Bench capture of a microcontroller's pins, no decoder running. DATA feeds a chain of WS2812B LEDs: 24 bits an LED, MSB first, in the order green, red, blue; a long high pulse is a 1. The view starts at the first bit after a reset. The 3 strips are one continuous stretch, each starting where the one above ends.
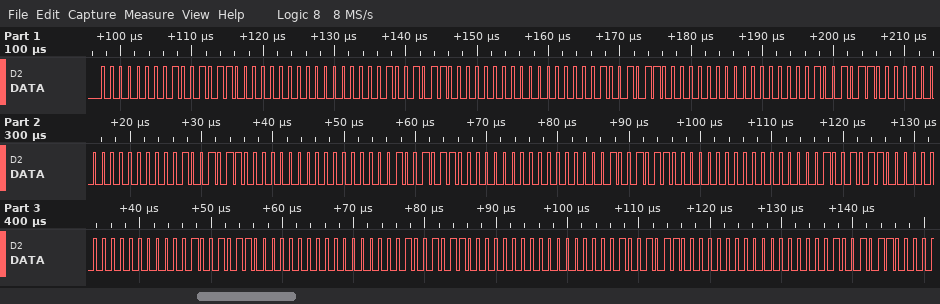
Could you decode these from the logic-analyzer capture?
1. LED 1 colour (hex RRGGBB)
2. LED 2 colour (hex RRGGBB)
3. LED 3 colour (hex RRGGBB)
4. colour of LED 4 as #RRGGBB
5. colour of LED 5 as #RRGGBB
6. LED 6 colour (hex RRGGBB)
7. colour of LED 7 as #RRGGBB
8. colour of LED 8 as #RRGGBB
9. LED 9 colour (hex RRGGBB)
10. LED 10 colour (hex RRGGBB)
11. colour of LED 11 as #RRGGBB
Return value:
#960000
#960000
#960000
#960000
#960000
#960000
#960000
#960000
#960000
#960000
#960000
